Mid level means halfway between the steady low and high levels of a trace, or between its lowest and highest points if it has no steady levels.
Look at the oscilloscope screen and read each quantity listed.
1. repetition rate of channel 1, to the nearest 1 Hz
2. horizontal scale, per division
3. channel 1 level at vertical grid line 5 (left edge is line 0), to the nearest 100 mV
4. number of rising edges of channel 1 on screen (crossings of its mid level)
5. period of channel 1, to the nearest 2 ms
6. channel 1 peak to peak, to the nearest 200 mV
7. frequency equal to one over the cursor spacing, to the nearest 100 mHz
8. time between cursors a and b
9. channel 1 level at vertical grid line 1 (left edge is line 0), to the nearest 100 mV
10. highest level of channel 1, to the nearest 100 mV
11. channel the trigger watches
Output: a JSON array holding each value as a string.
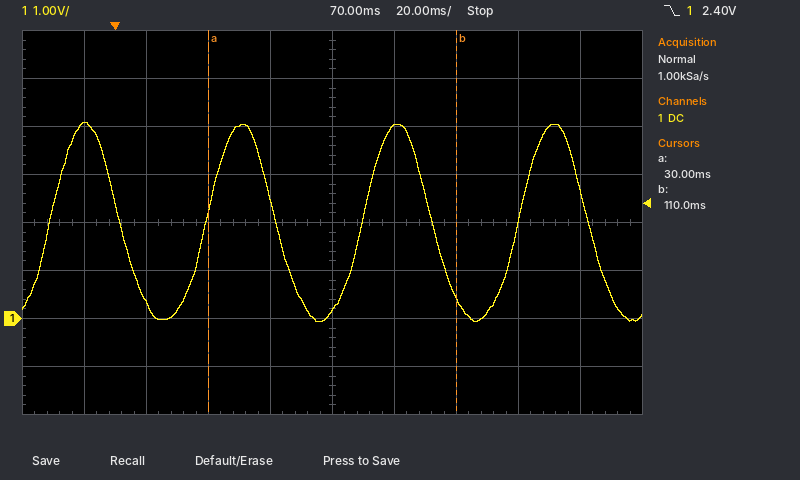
["20 Hz", "20 ms", "200 mV", "4", "50 ms", "4.2 V", "12.5 Hz", "80 ms", "4.1 V", "4.1 V", "channel 1"]
